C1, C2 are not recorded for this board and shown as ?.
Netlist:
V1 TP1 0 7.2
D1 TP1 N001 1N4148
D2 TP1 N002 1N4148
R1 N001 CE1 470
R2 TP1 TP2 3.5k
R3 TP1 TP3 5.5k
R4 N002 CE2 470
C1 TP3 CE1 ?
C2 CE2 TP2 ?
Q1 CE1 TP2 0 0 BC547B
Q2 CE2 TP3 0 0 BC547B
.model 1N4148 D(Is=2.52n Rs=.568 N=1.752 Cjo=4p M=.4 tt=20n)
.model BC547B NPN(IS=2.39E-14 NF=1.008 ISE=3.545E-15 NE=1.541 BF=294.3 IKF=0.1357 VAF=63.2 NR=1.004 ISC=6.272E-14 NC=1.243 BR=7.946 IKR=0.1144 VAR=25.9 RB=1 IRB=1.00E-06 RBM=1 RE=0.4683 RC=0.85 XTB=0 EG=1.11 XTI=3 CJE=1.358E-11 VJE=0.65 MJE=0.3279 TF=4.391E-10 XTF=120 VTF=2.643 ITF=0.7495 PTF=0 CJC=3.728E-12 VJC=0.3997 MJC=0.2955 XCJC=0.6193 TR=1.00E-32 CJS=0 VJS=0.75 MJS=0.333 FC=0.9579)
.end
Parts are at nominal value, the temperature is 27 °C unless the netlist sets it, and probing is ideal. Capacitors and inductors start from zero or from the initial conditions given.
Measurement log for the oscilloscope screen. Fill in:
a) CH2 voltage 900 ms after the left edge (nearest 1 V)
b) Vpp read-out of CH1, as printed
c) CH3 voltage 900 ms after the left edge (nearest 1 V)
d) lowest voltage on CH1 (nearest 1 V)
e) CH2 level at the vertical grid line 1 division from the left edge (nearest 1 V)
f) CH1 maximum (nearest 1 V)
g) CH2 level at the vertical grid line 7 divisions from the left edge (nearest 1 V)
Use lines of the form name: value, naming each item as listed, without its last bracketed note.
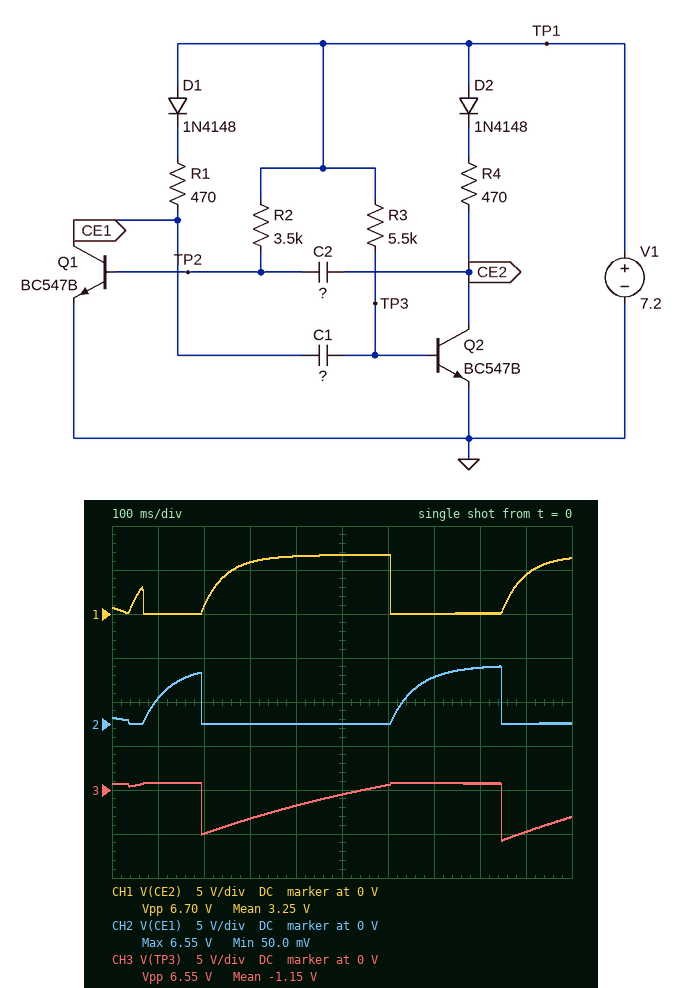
CH2 voltage 900 ms after the left edge: 0 V
Vpp read-out of CH1, as printed: 6.70 V
CH3 voltage 900 ms after the left edge: -5 V
lowest voltage on CH1: 0 V
CH2 level at the vertical grid line 1 division from the left edge: 3 V
CH1 maximum: 7 V
CH2 level at the vertical grid line 7 divisions from the left edge: 5 V
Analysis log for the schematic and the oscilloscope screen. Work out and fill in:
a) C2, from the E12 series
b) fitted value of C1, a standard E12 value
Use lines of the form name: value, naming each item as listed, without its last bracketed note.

C2, from the E12 series: 100 µF
fitted value of C1, a standard E12 value: 120 µF
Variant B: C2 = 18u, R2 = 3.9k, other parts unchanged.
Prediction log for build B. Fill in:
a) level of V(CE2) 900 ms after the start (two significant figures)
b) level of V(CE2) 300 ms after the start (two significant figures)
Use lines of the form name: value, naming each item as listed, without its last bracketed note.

level of V(CE2) 900 ms after the start: 6.7 V
level of V(CE2) 300 ms after the start: 6.8 V
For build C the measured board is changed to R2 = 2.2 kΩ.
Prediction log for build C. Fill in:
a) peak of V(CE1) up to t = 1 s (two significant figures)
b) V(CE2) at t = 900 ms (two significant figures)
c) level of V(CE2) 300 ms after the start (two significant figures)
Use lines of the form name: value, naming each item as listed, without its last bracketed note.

peak of V(CE1) up to t = 1 s: 6.1 V
V(CE2) at t = 900 ms: 6.5 V
level of V(CE2) 300 ms after the start: 6.2 V
